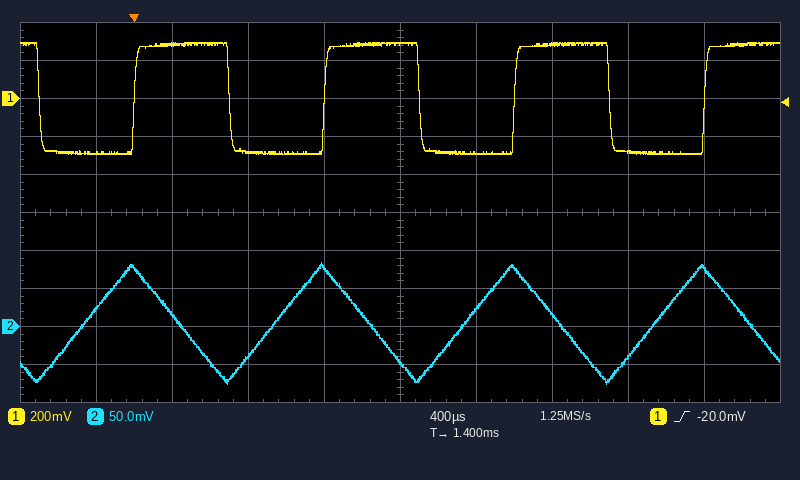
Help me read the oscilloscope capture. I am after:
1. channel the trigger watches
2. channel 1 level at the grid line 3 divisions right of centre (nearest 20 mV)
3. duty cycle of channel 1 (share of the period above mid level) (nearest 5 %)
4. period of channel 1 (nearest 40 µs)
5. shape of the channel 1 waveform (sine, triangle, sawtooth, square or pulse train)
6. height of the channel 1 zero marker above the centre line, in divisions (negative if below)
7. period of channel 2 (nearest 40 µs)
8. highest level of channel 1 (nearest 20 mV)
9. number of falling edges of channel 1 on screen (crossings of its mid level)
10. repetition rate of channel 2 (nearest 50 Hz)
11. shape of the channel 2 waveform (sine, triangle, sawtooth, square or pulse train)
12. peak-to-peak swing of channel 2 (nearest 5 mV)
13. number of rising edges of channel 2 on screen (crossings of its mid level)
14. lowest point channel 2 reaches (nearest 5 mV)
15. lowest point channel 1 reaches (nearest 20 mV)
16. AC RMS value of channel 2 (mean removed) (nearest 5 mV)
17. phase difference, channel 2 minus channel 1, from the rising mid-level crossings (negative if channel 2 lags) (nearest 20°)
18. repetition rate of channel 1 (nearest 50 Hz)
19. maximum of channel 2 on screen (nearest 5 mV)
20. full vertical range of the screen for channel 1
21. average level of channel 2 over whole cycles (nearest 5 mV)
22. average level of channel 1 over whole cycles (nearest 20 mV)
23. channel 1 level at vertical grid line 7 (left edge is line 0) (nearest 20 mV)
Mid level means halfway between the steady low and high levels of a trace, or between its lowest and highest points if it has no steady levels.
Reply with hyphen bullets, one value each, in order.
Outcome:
- channel 1
- -280 mV
- 50 %
- 1.00 ms
- square
- +3.0 div
- 1.00 ms
- 300 mV
- 4
- 1.00 kHz
- triangle
- 160 mV
- 4
- -75 mV
- -300 mV
- 45 mV
- +100°
- 1.00 kHz
- 85 mV
- 2 V
- 5 mV
- 0 mV
- 280 mV
